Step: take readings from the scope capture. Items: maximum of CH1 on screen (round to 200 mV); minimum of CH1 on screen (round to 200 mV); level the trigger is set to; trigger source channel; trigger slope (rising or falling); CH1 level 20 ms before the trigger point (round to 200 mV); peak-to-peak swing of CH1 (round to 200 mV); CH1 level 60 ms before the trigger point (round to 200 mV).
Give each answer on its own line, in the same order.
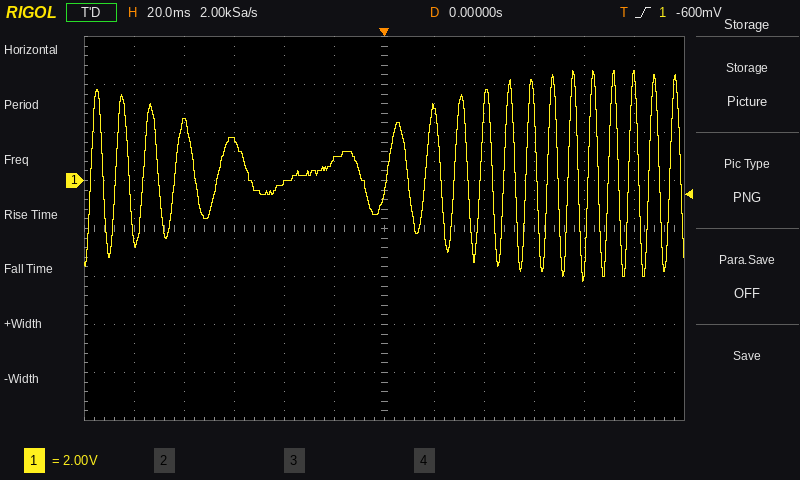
4.6 V
-4.2 V
-600 mV
CH1
rising
800 mV
8.8 V
1.6 V
